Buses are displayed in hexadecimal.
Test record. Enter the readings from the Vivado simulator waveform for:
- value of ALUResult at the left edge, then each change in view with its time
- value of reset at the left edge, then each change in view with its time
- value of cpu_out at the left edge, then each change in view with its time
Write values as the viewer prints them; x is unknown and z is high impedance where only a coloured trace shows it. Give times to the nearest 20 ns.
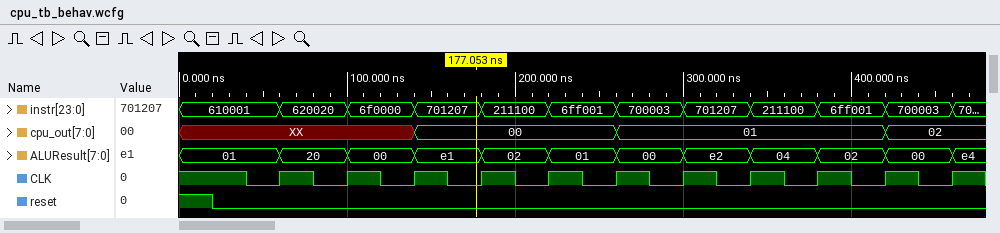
01, 20 at 60 ns, 00 at 100 ns, e1 at 140 ns, 02 at 180 ns, 01 at 220 ns, 00 at 260 ns, e2 at 300 ns, 04 at 340 ns, 02 at 380 ns, 00 at 420 ns, e4 at 460 ns
1, 0 at 20 ns
XX, 00 at 140 ns, 01 at 260 ns, 02 at 420 ns
